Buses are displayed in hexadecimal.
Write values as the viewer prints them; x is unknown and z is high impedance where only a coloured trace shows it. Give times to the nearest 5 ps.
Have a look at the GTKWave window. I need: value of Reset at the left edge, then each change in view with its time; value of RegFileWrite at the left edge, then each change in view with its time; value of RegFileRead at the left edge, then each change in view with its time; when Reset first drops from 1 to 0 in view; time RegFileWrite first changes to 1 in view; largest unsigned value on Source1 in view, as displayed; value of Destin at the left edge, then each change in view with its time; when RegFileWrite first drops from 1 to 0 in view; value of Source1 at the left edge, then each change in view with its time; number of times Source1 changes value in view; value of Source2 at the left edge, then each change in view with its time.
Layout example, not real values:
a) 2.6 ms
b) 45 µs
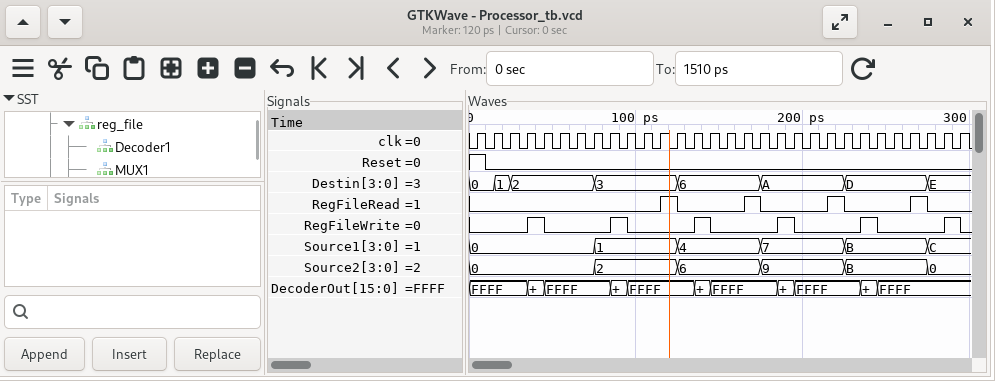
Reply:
a) 1, 0 at 10 ps
b) 0, 1 at 35 ps, 0 at 45 ps, 1 at 85 ps, 0 at 95 ps, 1 at 135 ps, 0 at 145 ps, 1 at 185 ps, 0 at 195 ps, 1 at 235 ps, 0 at 245 ps, 1 at 285 ps, 0 at 295 ps
c) 0, 1 at 115 ps, 0 at 125 ps, 1 at 165 ps, 0 at 175 ps, 1 at 215 ps, 0 at 225 ps, 1 at 265 ps, 0 at 275 ps
d) 10 ps
e) 35 ps
f) C
g) 0, 1 at 15 ps, 2 at 25 ps, 3 at 75 ps, 6 at 125 ps, A at 175 ps, D at 225 ps, E at 275 ps
h) 45 ps
i) 0, 1 at 75 ps, 4 at 125 ps, 7 at 175 ps, B at 225 ps, C at 275 ps
j) 5
k) 0, 2 at 75 ps, 6 at 125 ps, 9 at 175 ps, B at 225 ps, 0 at 275 ps
